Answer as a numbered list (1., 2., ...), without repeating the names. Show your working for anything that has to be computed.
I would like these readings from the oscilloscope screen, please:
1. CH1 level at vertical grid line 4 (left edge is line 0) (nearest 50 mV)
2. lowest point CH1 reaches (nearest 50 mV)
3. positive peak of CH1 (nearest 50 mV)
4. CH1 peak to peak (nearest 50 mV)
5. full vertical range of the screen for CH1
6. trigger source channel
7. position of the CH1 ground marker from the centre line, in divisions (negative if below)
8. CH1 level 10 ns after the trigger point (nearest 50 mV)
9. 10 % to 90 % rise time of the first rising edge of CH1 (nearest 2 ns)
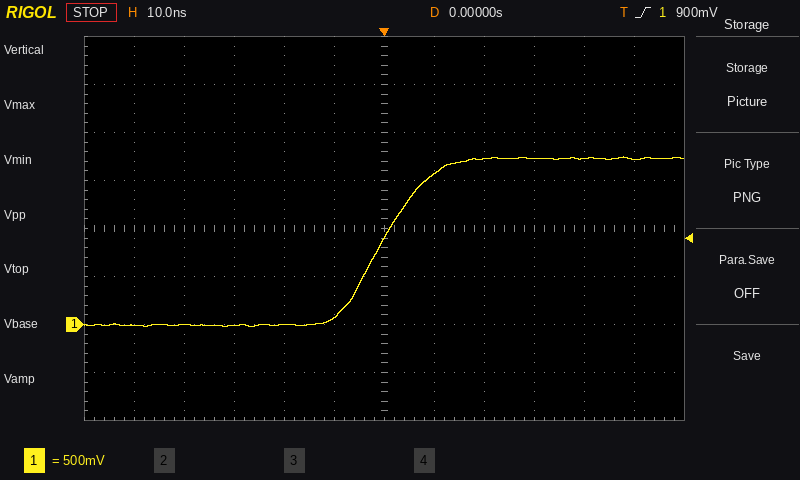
1. 0 mV
2. 0 mV
3. 1.75 V
4. 1.75 V − (0 mV) = 1.75 V
5. 4 V
6. CH1
7. -2.0 div
8. 1.55 V
9. 18 ns
